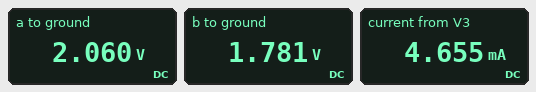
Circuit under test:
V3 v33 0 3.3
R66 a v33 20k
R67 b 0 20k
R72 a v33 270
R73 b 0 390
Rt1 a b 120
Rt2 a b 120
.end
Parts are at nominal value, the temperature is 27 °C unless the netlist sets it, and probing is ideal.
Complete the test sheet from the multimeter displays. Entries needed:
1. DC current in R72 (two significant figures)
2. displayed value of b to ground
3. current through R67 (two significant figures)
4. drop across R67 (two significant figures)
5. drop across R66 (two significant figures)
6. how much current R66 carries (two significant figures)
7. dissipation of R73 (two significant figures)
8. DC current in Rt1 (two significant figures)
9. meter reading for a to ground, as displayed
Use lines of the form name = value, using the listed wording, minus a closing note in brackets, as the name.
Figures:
DC current in R72 = 4.6 mA
displayed value of b to ground = 1.781 V
current through R67 = 89 µA
drop across R67 = 1.8 V
drop across R66 = 1.2 V
how much current R66 carries = 62 µA
dissipation of R73 = 8.1 mW
DC current in Rt1 = 2.3 mA
meter reading for a to ground, as displayed = 2.060 V
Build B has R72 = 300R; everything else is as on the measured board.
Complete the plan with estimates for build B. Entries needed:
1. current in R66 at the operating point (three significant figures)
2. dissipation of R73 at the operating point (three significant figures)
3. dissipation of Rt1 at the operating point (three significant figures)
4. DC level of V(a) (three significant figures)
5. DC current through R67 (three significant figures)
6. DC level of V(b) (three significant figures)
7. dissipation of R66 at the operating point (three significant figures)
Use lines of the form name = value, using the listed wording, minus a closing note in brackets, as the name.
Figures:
current in R66 at the operating point = 66.1 µA
dissipation of R73 at the operating point = 7.50 mW
dissipation of Rt1 at the operating point = 600 µW
DC level of V(a) = 1.98 V
DC current through R67 = 85.5 µA
DC level of V(b) = 1.71 V
dissipation of R66 at the operating point = 87.3 µW
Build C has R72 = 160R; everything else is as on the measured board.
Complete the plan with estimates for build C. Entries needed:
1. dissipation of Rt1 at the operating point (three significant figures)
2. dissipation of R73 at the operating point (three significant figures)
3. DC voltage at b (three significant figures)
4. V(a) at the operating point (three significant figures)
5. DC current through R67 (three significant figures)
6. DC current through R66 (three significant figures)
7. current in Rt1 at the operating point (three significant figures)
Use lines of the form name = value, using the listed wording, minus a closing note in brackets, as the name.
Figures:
dissipation of Rt1 at the operating point = 904 µW
dissipation of R73 at the operating point = 11.3 mW
DC voltage at b = 2.10 V
V(a) at the operating point = 2.43 V
DC current through R67 = 105 µA
DC current through R66 = 43.6 µA
current in Rt1 at the operating point = 2.74 mA
